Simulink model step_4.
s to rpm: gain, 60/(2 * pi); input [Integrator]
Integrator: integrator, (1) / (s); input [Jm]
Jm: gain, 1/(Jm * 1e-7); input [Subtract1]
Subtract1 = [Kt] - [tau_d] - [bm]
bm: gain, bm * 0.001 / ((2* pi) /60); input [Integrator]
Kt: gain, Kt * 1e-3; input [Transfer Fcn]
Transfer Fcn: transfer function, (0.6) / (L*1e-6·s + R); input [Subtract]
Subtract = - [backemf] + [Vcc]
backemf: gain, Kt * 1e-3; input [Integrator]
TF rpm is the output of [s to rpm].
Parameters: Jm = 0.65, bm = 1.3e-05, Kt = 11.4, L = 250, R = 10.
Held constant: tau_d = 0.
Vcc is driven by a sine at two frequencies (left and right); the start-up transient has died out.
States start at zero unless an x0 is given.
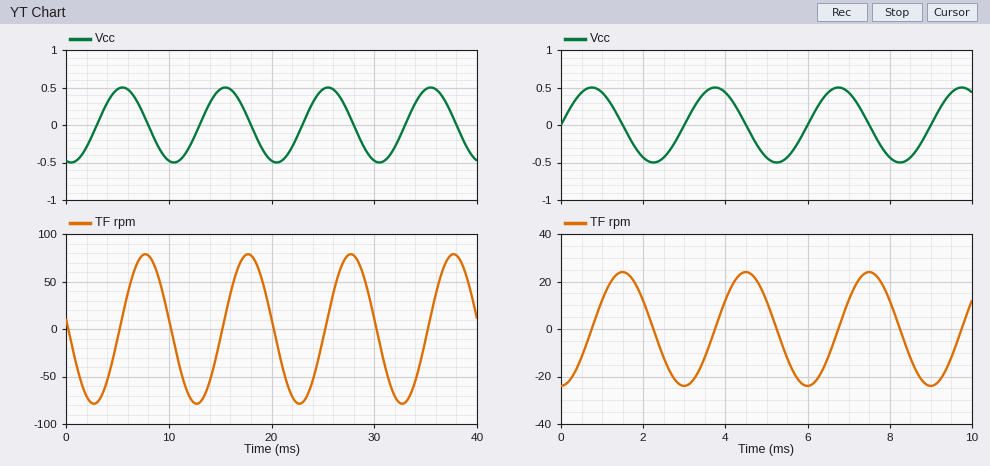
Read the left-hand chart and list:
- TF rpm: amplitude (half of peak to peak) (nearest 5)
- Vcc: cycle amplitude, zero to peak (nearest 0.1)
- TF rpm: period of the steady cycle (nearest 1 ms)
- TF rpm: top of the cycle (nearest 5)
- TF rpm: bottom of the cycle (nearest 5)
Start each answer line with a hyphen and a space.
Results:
- 80
- 0.5
- 10 ms
- 80
- -80
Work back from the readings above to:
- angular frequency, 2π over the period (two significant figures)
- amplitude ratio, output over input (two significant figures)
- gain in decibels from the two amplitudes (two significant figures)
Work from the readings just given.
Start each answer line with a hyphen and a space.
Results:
- 0.63 rad/ms
- 160
- 44 dB
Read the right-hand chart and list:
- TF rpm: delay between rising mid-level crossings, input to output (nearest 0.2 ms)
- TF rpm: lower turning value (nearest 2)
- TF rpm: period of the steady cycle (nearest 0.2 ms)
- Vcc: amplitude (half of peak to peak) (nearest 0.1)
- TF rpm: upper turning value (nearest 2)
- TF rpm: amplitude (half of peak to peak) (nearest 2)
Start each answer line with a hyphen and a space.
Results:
- 0.8 ms
- -24
- 3.0 ms
- 0.5
- 24
- 24
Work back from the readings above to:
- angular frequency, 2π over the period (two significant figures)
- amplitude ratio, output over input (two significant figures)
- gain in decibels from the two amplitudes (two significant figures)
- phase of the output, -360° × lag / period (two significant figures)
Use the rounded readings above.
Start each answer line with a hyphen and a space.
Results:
- 2.1 rad/ms
- 48
- 34 dB
- -96°
